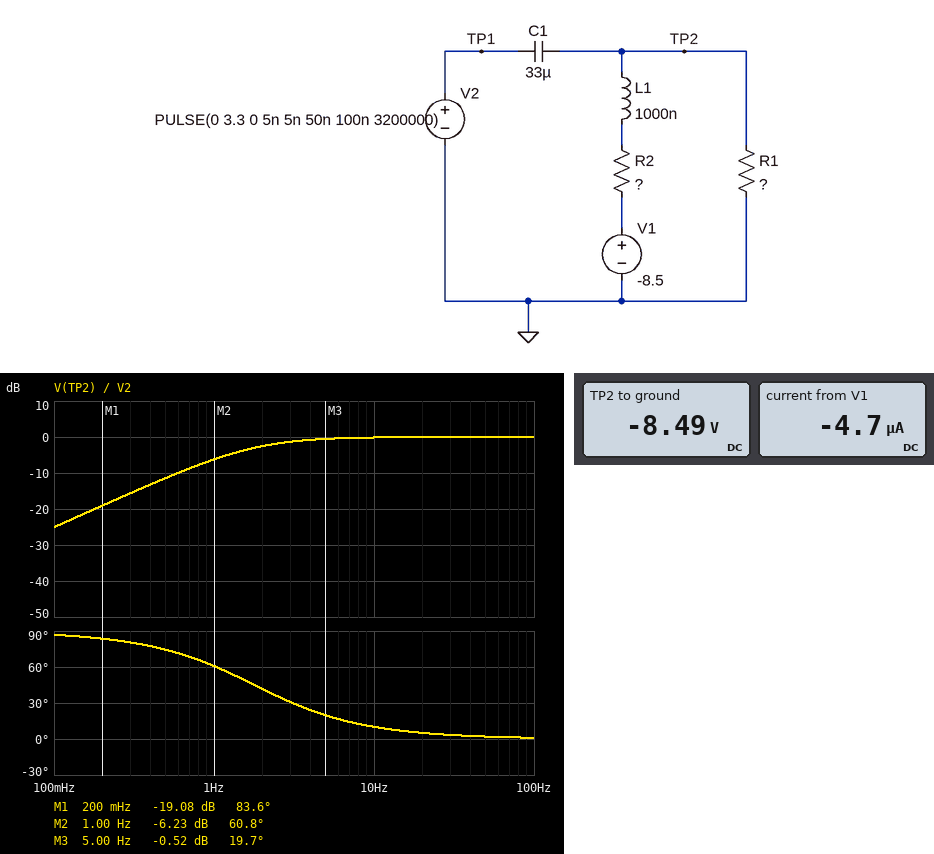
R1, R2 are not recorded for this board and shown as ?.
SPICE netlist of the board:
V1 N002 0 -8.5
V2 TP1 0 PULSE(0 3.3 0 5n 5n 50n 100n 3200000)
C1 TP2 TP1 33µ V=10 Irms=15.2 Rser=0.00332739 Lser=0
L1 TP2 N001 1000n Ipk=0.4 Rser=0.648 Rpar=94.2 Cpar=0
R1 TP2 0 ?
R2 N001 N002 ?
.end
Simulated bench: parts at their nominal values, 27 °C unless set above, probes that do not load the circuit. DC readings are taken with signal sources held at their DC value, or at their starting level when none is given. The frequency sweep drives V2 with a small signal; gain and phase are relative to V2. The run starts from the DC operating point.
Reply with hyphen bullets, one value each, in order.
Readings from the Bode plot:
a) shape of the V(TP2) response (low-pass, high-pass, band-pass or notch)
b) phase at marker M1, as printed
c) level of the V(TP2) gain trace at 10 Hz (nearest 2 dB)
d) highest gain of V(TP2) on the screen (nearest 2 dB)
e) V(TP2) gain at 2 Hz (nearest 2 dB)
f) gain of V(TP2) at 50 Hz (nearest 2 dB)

- high-pass
- 83.6 deg
- 0 dB
- 0 dB
- -2 dB
- 0 dB
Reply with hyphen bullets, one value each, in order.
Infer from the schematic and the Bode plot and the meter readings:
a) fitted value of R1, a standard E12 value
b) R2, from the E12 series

- 1.8 MΩ
- 2.7 kΩ
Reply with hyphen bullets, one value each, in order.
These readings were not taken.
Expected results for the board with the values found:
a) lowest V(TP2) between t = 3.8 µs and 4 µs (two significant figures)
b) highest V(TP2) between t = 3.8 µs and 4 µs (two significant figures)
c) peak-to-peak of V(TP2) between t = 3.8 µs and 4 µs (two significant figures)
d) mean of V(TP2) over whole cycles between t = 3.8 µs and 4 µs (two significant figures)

- -8.5 V
- -5.2 V
- 3.3 V
- -6.7 V
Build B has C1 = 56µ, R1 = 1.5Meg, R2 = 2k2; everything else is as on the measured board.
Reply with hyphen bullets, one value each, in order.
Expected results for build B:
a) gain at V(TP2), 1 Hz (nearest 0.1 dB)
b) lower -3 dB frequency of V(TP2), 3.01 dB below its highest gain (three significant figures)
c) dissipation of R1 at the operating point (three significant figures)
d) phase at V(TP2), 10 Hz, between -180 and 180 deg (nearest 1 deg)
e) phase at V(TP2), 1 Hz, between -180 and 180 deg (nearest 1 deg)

- -4.3 dB
- 1.29 Hz
- 48.0 µW
- 7 deg
- 52 deg
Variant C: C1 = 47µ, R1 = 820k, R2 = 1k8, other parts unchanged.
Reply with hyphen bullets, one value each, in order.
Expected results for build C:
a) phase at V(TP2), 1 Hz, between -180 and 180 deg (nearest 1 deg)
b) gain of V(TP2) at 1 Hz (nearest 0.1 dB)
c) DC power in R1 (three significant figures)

- 62 deg
- -6.6 dB
- 87.7 µW
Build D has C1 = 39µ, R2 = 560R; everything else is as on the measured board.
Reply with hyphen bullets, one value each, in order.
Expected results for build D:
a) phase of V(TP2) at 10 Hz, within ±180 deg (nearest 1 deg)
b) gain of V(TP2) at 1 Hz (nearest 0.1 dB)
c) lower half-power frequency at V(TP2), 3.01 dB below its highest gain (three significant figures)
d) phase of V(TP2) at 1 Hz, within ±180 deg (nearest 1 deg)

- 36 deg
- -17.3 dB
- 7.28 Hz
- 82 deg
